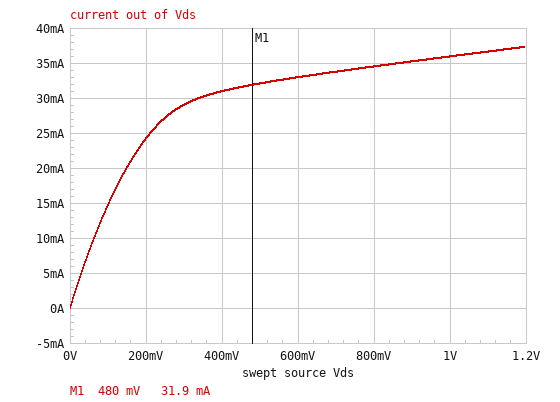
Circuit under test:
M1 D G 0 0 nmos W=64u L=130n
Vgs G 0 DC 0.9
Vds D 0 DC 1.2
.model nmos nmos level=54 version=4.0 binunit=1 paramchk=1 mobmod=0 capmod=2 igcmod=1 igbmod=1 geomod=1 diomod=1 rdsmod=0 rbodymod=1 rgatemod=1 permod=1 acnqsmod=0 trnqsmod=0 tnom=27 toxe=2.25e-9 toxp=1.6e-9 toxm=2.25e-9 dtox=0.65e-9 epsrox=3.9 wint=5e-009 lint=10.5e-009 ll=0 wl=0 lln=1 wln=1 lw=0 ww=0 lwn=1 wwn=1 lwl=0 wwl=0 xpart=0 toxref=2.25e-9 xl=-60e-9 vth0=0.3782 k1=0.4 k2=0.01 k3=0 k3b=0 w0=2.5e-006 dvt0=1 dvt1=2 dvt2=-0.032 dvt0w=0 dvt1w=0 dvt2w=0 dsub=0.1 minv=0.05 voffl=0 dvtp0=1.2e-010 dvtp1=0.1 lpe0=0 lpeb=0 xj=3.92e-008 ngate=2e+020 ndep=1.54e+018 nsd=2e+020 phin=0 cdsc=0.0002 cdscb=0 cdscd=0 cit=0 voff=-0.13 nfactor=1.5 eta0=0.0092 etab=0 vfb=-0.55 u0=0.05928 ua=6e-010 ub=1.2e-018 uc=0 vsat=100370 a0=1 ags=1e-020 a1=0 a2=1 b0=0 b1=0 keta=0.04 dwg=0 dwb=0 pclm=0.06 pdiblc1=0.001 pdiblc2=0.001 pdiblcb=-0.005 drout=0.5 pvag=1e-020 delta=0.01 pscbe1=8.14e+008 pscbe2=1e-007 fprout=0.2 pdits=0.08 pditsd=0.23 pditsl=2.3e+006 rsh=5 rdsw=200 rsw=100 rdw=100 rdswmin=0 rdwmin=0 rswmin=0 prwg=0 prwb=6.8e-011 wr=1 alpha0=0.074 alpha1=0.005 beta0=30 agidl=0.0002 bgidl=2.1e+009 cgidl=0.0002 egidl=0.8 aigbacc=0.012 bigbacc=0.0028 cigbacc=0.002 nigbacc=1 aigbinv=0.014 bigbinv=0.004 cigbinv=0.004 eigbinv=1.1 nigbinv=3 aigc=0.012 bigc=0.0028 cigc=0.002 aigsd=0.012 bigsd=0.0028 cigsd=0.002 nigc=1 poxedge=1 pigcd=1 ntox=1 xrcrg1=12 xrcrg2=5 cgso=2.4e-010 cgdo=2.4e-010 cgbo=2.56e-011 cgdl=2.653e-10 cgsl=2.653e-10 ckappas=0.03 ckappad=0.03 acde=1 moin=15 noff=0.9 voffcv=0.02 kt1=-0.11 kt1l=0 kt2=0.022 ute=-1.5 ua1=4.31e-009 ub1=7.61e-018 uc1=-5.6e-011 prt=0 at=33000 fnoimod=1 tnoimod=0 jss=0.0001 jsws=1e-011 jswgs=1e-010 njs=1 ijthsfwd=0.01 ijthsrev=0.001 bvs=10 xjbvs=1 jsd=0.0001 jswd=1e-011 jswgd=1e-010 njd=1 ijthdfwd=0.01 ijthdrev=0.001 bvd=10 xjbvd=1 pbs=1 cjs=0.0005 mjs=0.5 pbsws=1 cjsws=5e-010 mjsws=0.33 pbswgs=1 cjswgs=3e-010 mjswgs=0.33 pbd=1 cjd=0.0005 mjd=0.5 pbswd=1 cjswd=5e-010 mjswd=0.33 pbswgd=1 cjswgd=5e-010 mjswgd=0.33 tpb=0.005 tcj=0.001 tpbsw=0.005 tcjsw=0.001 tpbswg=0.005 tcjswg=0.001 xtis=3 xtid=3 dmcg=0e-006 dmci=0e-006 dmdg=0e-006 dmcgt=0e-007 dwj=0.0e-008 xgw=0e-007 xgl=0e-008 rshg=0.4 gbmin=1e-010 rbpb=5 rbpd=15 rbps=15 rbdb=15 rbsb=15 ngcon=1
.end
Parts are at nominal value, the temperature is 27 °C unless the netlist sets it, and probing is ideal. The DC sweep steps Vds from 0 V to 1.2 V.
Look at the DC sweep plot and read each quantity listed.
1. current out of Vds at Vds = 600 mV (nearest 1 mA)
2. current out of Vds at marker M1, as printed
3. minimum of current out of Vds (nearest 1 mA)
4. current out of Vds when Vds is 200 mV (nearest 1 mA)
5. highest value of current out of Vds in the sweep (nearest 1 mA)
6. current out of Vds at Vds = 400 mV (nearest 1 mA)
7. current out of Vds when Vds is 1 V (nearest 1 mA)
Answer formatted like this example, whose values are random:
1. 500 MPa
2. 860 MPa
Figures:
1. 33 mA
2. 31.9 mA
3. 0 A
4. 24 mA
5. 37 mA
6. 31 mA
7. 36 mA
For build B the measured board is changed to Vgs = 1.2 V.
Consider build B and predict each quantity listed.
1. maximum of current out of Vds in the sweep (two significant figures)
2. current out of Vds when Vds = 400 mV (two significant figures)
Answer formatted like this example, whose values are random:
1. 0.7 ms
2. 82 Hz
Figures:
1. 57 mA
2. 47 mA
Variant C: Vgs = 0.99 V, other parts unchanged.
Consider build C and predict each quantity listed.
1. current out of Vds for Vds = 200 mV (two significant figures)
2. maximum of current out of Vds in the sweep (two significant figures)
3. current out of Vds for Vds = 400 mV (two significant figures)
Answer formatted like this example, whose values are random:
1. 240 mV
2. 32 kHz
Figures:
1. 27 mA
2. 43 mA
3. 36 mA
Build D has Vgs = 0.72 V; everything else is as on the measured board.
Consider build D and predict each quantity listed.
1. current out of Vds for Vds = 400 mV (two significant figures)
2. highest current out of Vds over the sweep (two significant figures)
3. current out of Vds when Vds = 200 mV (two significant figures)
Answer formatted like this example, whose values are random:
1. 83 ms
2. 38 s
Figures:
1. 20 mA
2. 25 mA
3. 17 mA
